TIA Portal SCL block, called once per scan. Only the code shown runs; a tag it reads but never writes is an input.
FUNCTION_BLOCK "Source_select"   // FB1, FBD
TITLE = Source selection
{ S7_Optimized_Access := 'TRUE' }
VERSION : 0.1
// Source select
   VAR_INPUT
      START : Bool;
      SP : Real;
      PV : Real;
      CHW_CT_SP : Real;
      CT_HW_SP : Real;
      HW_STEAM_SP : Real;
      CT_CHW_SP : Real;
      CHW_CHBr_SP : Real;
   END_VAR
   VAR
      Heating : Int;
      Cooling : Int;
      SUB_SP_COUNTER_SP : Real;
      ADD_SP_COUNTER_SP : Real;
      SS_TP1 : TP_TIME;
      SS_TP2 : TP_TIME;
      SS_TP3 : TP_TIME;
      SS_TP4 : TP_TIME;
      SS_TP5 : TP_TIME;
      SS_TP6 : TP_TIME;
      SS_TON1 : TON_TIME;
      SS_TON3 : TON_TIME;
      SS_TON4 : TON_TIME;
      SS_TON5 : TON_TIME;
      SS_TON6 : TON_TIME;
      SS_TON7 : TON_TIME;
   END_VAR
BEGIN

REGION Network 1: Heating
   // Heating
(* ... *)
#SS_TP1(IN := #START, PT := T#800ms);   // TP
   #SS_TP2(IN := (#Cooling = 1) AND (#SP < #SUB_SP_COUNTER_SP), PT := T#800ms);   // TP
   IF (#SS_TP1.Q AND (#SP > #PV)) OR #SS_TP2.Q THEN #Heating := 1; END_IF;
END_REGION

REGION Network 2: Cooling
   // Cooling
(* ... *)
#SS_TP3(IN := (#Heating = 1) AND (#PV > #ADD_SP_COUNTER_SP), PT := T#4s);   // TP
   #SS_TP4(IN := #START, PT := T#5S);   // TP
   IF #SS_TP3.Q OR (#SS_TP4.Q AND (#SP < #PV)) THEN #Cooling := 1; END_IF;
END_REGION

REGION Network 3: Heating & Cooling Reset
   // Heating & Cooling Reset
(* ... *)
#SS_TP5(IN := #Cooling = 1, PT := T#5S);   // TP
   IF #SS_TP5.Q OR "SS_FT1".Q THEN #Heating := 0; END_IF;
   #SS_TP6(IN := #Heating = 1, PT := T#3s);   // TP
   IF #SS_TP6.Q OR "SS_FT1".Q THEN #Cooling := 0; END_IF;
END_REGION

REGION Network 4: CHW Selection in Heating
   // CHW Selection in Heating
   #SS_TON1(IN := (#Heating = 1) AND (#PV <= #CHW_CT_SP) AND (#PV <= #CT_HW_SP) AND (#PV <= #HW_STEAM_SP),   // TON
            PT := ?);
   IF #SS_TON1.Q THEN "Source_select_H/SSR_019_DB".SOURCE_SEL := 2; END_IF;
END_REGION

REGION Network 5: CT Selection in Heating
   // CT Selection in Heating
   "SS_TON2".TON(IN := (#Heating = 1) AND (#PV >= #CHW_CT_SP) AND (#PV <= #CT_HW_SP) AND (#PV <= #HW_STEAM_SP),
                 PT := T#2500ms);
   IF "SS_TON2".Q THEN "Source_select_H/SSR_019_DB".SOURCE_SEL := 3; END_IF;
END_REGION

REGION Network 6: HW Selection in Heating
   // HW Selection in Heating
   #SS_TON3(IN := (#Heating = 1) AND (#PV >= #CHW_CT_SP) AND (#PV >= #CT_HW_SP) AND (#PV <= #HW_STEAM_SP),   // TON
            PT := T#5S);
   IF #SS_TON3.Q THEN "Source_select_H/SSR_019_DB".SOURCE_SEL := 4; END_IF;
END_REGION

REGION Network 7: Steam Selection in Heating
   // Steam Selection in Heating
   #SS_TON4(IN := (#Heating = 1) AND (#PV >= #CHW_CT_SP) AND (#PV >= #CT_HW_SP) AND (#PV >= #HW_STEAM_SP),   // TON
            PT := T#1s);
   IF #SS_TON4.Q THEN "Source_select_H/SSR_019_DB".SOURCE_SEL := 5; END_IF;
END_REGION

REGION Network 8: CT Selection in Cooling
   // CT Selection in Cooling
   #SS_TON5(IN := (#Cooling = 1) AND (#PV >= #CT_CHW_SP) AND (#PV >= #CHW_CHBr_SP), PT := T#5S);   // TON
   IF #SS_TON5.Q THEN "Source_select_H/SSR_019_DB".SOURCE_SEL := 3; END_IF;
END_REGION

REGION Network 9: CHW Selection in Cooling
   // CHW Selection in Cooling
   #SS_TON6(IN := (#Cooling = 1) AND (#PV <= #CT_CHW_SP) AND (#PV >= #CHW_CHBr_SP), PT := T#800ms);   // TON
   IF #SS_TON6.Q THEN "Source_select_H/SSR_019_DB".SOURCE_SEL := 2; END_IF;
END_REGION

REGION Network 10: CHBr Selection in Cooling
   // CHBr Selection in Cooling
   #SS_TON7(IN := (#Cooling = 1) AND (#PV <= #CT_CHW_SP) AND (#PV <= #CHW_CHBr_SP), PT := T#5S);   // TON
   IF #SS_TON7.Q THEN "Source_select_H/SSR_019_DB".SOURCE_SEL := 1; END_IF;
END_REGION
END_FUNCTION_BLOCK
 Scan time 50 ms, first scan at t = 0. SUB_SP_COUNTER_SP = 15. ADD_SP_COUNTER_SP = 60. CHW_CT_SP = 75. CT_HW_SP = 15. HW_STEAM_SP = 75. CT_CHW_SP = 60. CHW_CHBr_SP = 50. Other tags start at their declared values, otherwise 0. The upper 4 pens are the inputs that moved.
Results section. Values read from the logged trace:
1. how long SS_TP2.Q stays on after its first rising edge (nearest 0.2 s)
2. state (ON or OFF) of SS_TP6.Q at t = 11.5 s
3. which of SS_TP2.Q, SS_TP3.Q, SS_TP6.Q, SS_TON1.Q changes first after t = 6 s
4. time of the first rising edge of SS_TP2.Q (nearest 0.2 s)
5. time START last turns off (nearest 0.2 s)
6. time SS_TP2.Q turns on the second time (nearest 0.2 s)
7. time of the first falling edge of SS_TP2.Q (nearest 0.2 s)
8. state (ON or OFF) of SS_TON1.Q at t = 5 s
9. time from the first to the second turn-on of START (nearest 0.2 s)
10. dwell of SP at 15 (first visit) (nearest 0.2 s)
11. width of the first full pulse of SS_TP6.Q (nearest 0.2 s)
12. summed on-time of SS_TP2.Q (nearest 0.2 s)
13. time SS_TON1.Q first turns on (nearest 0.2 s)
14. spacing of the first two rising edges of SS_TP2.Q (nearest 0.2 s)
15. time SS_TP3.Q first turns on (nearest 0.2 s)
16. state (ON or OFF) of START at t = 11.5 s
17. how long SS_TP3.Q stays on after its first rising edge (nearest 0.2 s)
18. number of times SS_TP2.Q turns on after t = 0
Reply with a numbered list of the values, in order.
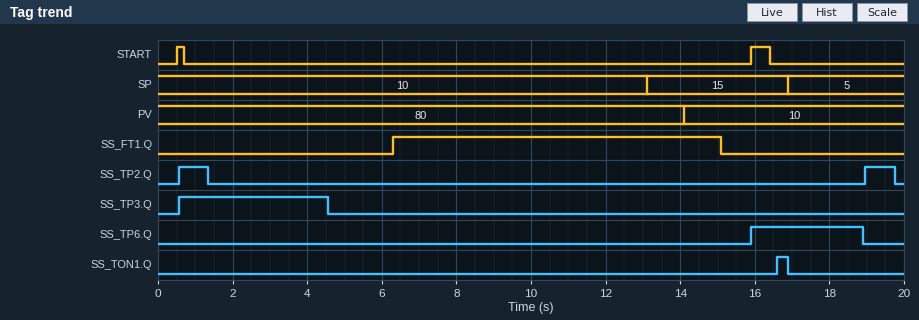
1. 0.8 s
2. OFF
3. SS_TP6.Q
4. 0.6 s
5. 16.4 s
6. 19.0 s
7. 1.4 s
8. OFF
9. 15.4 s
10. 3.8 s
11. 3.0 s
12. 1.6 s
13. 16.6 s
14. 18.4 s
15. 0.6 s
16. OFF
17. 4.0 s
18. 2
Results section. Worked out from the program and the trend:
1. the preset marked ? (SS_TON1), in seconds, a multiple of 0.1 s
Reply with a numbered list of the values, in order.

1. 0.7 s
